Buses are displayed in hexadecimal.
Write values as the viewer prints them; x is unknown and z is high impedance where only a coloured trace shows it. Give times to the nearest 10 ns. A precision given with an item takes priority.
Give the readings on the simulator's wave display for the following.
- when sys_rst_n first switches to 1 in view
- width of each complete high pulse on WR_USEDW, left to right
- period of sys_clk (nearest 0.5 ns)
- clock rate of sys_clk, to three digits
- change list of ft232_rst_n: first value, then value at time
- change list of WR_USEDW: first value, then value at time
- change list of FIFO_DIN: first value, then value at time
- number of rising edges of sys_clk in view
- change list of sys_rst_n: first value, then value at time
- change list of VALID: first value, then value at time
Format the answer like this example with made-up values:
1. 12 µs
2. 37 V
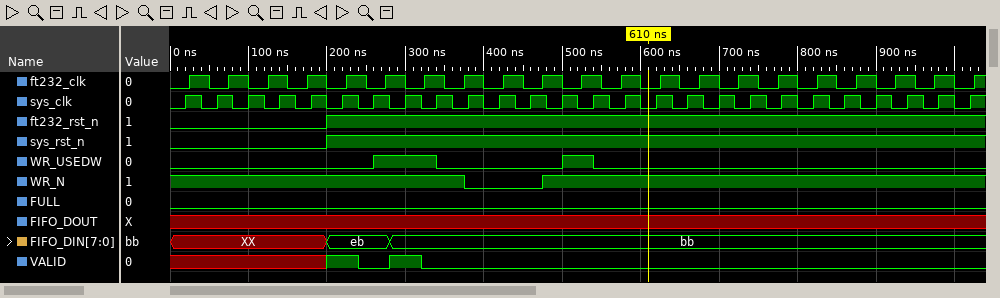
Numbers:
1. 200 ns
2. 80 ns, 40 ns
3. 40 ns
4. 25.0 MHz
5. 0, 1 at 200 ns
6. 0, 1 at 260 ns, 0 at 340 ns, 1 at 500 ns, 0 at 540 ns
7. XX, eb at 200 ns, bb at 280 ns
8. 26
9. 0, 1 at 200 ns
10. x, 1 at 200 ns, 0 at 240 ns, 1 at 280 ns, 0 at 320 ns
